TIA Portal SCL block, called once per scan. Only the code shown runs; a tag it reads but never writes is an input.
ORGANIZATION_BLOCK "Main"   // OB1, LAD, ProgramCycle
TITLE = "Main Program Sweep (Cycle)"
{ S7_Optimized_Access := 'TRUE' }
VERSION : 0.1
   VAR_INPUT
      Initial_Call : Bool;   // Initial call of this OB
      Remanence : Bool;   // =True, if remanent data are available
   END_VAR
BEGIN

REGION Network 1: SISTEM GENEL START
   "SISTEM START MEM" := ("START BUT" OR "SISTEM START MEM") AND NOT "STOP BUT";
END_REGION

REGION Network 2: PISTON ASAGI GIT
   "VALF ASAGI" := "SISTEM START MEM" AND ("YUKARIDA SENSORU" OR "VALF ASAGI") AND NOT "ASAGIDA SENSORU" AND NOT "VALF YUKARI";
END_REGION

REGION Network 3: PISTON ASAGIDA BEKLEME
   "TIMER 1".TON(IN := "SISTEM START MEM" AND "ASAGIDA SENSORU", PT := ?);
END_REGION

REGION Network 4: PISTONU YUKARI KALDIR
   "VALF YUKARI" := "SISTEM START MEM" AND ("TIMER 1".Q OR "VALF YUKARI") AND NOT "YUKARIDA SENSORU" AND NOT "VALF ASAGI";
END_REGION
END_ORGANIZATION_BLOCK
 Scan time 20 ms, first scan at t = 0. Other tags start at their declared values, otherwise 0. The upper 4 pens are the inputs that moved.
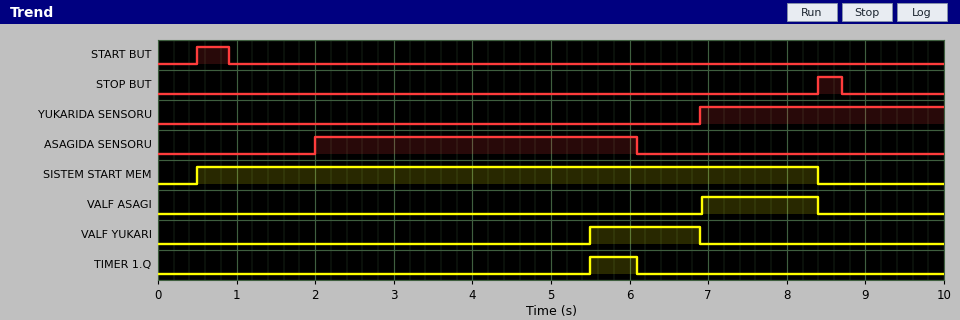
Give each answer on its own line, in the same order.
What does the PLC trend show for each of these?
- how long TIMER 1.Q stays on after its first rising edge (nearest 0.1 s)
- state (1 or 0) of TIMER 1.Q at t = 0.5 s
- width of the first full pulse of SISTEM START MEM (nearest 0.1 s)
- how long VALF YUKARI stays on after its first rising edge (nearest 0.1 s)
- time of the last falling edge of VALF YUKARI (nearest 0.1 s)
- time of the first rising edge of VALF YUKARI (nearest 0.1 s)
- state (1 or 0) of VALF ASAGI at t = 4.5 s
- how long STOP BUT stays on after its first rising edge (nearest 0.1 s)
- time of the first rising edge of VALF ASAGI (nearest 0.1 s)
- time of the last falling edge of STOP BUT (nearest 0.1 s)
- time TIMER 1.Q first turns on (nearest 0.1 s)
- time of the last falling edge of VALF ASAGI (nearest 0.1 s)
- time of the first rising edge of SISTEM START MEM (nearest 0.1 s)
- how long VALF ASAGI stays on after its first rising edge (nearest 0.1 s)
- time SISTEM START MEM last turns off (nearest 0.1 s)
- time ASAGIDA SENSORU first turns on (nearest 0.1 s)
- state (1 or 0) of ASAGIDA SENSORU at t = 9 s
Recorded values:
0.6 s
0
7.9 s
1.4 s
6.9 s
5.5 s
0
0.3 s
6.9 s
8.7 s
5.5 s
8.4 s
0.5 s
1.5 s
8.4 s
2.0 s
0
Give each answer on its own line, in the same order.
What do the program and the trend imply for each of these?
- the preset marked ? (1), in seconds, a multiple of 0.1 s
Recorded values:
3.5 s
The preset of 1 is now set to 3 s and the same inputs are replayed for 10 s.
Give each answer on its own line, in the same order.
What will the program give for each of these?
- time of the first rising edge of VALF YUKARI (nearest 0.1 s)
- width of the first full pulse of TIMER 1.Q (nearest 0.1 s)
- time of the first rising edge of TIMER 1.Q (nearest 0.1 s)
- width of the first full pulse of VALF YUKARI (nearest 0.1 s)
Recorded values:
5.0 s
1.1 s
5.0 s
1.9 s
